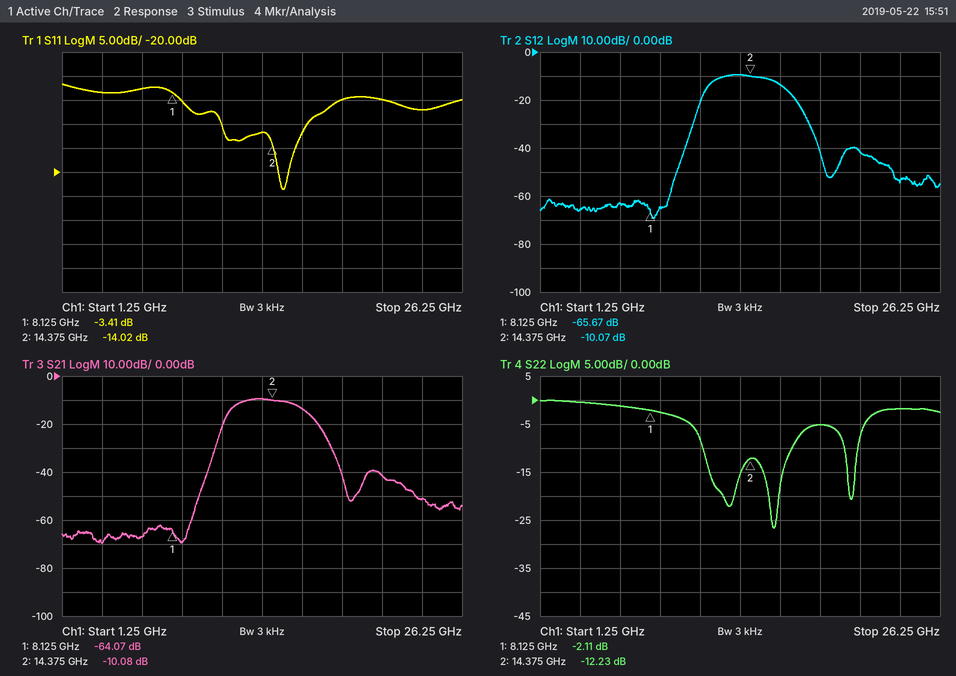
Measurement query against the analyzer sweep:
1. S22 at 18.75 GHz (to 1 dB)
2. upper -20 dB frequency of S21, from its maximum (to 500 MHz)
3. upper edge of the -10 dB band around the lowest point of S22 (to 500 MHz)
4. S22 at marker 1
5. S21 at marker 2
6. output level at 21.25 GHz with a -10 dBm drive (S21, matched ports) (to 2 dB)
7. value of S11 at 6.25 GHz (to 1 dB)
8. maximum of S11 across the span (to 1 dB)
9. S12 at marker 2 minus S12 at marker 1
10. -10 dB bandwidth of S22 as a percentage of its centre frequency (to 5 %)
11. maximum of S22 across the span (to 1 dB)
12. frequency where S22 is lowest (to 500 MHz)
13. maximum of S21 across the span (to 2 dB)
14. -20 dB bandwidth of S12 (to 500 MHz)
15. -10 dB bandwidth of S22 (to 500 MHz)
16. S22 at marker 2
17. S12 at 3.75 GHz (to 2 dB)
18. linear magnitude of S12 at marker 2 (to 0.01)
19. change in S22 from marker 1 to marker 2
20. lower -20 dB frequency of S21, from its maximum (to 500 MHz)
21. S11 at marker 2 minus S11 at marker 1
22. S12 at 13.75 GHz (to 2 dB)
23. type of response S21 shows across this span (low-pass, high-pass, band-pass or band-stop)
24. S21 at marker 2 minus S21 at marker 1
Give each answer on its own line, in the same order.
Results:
-5 dB
18.0 GHz
17.0 GHz
-2.11 dB
-10.08 dB
-52 dBm
-3 dB
-2 dB
55.60 dB
40 %
0 dB
16.0 GHz
-10 dB
7.0 GHz
5.5 GHz
-12.23 dB
-66 dB
0.31
-10.12 dB
11.0 GHz
-10.61 dB
-10 dB
band-pass
53.99 dB
